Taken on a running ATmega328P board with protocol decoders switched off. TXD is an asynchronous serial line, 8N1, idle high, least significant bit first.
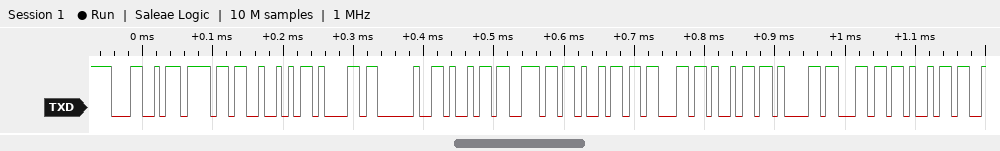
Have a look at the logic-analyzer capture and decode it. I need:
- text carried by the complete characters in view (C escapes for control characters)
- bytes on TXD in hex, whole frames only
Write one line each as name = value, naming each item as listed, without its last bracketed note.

text carried by the complete characters in view = "LoRa iniciali"
bytes on TXD in hex, whole frames only = 0x4C 0x6F 0x52 0x61 0x20 0x69 0x6E 0x69 0x63 0x69 0x61 0x6C 0x69
